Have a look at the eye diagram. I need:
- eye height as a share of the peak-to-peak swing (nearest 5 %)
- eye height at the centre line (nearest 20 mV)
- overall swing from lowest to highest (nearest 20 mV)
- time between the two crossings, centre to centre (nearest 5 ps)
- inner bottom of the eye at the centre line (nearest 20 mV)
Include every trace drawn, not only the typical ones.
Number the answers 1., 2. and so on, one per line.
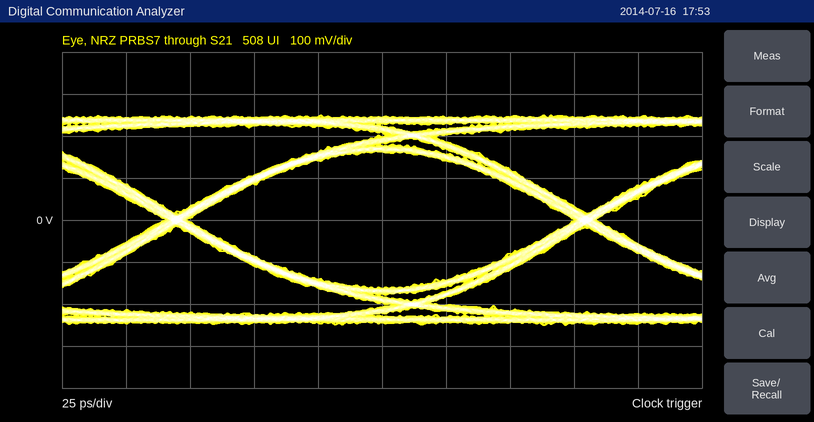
1. 65 %
2. 320 mV
3. 500 mV
4. 160 ps
5. -160 mV
